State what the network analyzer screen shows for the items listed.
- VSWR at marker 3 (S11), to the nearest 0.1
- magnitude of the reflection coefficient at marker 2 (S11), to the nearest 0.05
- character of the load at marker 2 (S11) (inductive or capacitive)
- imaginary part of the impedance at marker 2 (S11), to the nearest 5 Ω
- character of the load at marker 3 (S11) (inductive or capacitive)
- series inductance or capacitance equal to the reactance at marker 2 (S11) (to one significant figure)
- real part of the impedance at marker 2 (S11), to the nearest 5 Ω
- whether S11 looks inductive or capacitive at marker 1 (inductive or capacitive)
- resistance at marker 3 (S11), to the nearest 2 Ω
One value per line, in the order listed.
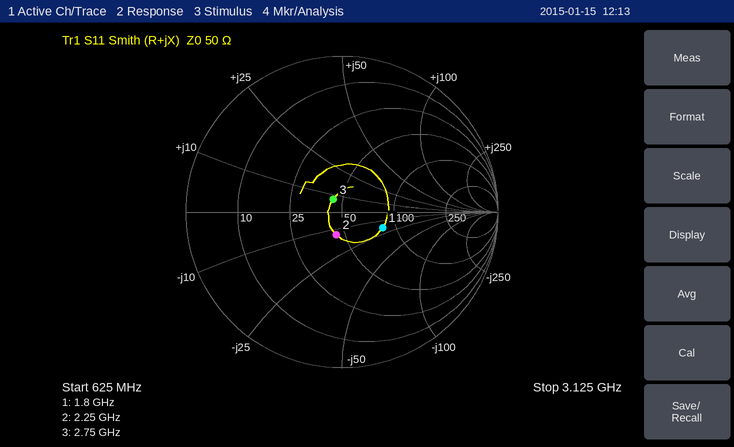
1.2
0.15
capacitive
-15 Ω
inductive
5 pF
45 Ω
capacitive
44 Ω
